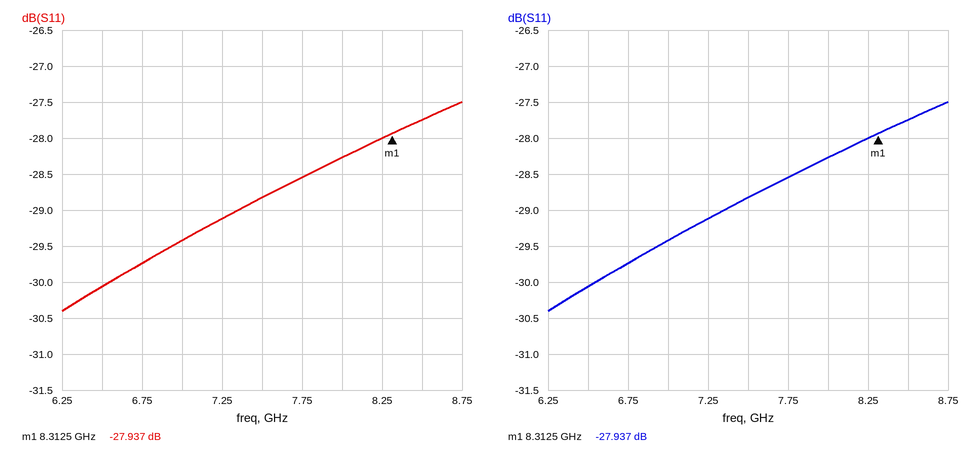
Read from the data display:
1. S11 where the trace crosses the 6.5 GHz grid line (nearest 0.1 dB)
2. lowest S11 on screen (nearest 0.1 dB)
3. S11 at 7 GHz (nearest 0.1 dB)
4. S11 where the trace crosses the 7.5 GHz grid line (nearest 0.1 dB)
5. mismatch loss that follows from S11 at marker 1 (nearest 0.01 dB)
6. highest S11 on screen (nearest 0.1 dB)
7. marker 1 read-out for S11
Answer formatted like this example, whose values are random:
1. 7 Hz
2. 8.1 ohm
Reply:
1. -30.1 dB
2. -30.4 dB
3. -29.4 dB
4. -28.8 dB
5. 0.01 dB
6. -27.5 dB
7. -27.937 dB
